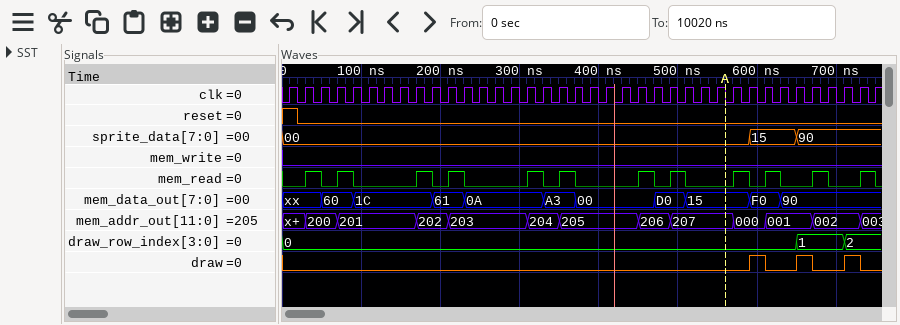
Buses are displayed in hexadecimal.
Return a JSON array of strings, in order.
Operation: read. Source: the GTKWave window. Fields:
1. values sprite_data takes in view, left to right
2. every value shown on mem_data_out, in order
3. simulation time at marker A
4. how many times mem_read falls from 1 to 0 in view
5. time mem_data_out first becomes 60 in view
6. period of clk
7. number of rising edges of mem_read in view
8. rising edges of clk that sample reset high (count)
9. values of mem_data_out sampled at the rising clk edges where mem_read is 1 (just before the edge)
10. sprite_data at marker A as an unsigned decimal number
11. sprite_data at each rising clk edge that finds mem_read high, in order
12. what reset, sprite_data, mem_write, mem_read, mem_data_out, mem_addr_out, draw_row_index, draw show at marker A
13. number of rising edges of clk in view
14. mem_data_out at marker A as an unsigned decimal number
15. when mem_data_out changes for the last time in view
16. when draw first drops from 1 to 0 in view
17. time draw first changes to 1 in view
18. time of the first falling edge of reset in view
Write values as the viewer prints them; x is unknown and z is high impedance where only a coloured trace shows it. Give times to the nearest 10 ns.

["00, 15, 90", "xx, 60, 1C, 61, 0A, A3, 00, D0, 15, F0, 90", "560 ns", "12", "50 ns", "20 ns", "12", "1", "xx, 60, 1C, 61, 0A, A3, 00, D0, 15, F0, 90, 90", "0", "00, 00, 00, 00, 00, 00, 00, 00, 00, 15, 90, 90", "reset=0, sprite_data=00, mem_write=0, mem_read=0, mem_data_out=15, mem_addr_out=207, draw_row_index=0, draw=0", "38", "21", "630 ns", "610 ns", "590 ns", "20 ns"]
